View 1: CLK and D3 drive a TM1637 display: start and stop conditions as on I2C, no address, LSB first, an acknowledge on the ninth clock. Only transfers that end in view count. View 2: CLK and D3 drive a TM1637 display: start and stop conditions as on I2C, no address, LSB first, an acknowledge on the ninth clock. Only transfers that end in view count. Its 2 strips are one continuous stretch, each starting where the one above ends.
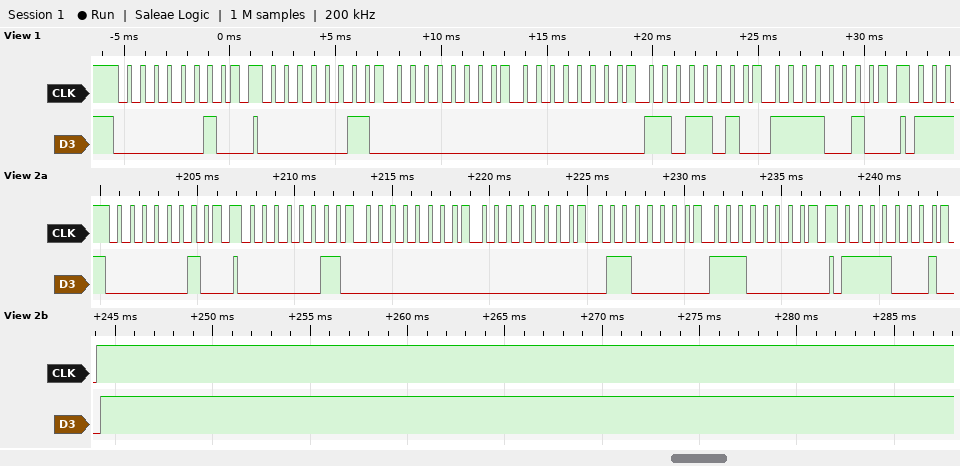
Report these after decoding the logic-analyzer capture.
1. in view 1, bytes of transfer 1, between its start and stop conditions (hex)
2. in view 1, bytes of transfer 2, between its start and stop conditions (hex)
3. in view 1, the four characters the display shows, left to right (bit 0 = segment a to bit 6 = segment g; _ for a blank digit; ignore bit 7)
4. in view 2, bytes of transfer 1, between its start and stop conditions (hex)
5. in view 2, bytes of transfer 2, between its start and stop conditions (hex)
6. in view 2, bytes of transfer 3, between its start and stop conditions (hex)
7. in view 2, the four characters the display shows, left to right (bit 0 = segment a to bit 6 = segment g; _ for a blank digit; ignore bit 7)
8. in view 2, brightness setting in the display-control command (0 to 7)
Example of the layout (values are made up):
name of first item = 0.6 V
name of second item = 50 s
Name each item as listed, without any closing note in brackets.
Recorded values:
in view 1, bytes of transfer 1, between its start and stop conditions = 40
in view 1, bytes of transfer 2, between its start and stop conditions = C0 00 00 5B 4F
in view 1, the four characters the display shows, left to right = __23
in view 2, bytes of transfer 1, between its start and stop conditions = 40
in view 2, bytes of transfer 2, between its start and stop conditions = C0 00 00 06 07
in view 2, bytes of transfer 3, between its start and stop conditions = 8F
in view 2, the four characters the display shows, left to right = __17
in view 2, brightness setting in the display-control command = 7
